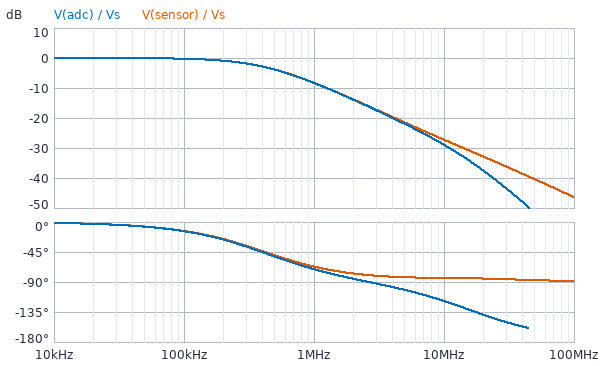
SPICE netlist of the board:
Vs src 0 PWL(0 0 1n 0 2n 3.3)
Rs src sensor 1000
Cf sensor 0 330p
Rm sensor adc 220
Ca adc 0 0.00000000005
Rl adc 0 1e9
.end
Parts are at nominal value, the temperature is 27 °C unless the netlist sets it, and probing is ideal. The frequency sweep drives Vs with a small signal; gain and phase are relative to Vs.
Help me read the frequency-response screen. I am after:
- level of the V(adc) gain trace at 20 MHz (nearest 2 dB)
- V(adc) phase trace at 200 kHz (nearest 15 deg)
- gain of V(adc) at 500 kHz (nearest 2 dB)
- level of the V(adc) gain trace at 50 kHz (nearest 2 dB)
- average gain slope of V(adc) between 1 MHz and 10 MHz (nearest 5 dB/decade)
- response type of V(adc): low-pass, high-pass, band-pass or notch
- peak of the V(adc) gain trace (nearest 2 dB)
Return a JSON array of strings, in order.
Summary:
["-38 dB", "-30 deg", "-4 dB", "0 dB", "-20 dB/decade", "low-pass", "0 dB"]
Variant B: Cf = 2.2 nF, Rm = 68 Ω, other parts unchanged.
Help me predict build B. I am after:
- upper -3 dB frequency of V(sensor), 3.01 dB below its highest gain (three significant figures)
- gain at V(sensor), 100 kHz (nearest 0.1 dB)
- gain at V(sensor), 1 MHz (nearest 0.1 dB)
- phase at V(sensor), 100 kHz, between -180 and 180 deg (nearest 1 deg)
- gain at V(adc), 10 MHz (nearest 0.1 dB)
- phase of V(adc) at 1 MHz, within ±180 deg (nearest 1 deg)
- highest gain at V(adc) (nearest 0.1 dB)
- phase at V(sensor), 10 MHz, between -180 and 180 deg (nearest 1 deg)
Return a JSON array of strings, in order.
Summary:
["70.7 kHz", "-4.8 dB", "-23.0 dB", "-55 deg", "-43.2 dB", "-87 deg", "0 dB", "-89 deg"]
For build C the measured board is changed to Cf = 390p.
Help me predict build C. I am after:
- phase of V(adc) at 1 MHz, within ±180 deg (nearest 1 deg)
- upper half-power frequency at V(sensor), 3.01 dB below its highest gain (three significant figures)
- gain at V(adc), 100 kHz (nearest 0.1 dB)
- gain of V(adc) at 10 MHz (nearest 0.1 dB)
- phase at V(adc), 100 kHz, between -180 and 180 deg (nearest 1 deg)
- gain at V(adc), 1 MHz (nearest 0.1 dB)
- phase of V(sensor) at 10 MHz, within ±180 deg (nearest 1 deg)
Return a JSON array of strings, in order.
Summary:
["-74 deg", "361 kHz", "-0.3 dB", "-30.2 dB", "-16 deg", "-9.4 dB", "-85 deg"]
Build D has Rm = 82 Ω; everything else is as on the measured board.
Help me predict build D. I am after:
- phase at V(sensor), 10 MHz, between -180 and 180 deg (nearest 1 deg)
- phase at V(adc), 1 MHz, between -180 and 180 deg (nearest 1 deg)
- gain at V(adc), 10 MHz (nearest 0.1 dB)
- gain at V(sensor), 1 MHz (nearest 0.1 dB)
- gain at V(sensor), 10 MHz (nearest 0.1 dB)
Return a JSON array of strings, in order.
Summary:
["-86 deg", "-69 deg", "-27.8 dB", "-8.3 dB", "-27.5 dB"]
